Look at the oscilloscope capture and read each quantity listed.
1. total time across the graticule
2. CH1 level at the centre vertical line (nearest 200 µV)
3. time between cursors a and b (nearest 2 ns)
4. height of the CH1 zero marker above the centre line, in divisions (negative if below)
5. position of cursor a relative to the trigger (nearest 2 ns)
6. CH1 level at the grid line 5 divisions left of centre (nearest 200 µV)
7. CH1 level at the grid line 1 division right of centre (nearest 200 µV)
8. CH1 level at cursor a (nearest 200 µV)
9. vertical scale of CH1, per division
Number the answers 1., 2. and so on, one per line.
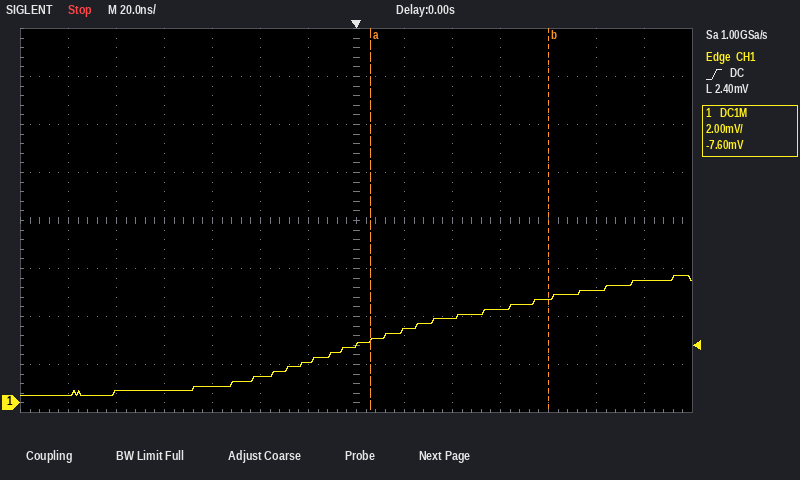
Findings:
1. 280 ns
2. 2.4 mV
3. 74 ns
4. -3.8 div
5. +6 ns
6. 400 µV
7. 3.0 mV
8. 2.6 mV
9. 2 mV
